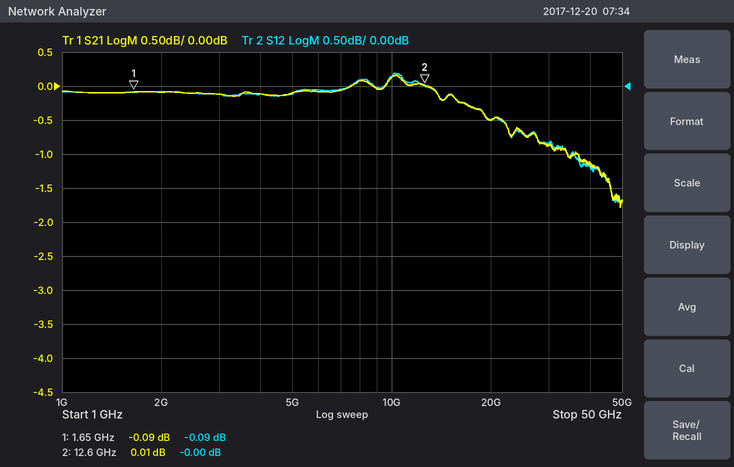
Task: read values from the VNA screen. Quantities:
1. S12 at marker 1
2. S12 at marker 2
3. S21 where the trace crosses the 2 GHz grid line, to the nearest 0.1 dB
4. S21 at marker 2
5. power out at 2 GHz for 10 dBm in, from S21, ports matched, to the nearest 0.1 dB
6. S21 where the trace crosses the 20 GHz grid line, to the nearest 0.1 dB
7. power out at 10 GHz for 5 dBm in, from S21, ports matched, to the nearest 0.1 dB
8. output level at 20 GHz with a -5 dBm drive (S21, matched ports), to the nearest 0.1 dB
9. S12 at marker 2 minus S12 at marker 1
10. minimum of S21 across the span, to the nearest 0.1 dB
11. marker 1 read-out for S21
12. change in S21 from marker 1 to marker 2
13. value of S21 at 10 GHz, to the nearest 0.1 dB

-0.09 dB
-0.00 dB
-0.1 dB
0.01 dB
9.9 dBm
-0.5 dB
5.1 dBm
-5.5 dBm
0.09 dB
-1.8 dB
-0.09 dB
0.10 dB
0.1 dB
